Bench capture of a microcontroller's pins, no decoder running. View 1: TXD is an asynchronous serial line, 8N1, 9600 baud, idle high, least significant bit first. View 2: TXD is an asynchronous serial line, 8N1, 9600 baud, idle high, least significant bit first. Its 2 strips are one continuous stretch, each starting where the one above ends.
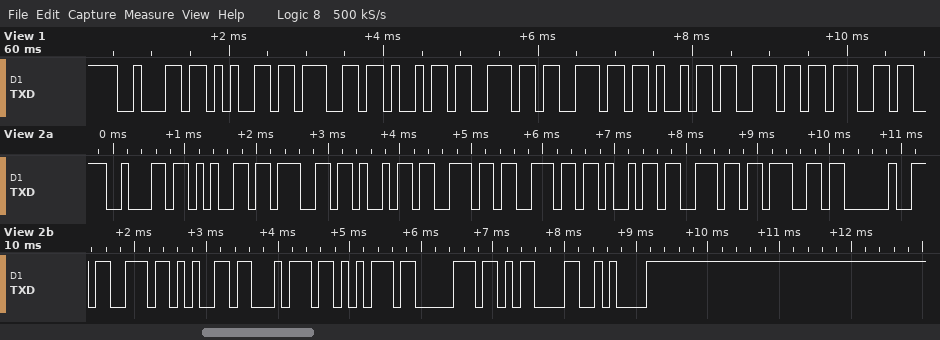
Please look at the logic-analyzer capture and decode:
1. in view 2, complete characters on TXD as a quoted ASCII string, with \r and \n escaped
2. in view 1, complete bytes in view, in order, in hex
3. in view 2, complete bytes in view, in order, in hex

"beginning setup\r\n"
0x62 0x65 0x67 0x69 0x6E 0x6E 0x69 0x6E 0x67
62 65 67 69 6E 6E 69 6E 67 20 73 65 74 75 70 0D 0A
